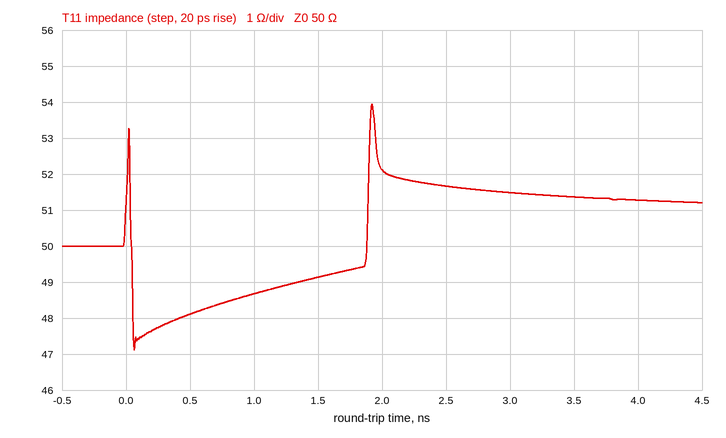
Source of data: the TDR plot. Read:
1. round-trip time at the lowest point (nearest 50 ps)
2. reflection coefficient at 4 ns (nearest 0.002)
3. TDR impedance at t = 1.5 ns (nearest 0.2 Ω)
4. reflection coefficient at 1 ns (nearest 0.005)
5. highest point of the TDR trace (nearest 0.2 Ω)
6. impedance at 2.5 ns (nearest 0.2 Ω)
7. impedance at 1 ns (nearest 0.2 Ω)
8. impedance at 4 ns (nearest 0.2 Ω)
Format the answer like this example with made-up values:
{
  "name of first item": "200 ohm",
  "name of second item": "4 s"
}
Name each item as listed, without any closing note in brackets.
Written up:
{
  "round-trip time at the lowest point": "50 ps",
  "reflection coefficient at 4 ns": "+0.012",
  "TDR impedance at t = 1.5 ns": "49.2 Ω",
  "reflection coefficient at 1 ns": "-0.015",
  "highest point of the TDR trace": "54.0 Ω",
  "impedance at 2.5 ns": "51.6 Ω",
  "impedance at 1 ns": "48.6 Ω",
  "impedance at 4 ns": "51.2 Ω"
}
